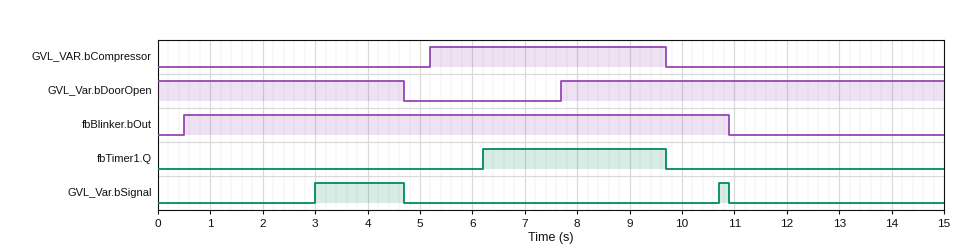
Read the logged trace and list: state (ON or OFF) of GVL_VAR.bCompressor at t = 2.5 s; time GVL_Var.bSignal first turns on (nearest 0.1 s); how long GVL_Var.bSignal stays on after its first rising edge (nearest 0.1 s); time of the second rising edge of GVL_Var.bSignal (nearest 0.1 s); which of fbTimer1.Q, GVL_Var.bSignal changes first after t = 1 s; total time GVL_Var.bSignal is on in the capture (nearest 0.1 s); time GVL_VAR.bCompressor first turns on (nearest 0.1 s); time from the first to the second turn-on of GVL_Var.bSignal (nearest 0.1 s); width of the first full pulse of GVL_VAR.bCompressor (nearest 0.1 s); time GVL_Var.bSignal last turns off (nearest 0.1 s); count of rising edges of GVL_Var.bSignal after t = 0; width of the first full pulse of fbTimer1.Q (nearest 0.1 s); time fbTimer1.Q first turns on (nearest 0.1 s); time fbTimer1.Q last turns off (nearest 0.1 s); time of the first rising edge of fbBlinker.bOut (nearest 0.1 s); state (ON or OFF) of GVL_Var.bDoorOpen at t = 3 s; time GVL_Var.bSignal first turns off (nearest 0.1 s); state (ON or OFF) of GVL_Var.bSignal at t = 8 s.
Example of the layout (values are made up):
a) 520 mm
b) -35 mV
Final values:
a) OFF
b) 3.0 s
c) 1.7 s
d) 10.7 s
e) GVL_Var.bSignal
f) 1.9 s
g) 5.2 s
h) 7.7 s
i) 4.5 s
j) 10.9 s
k) 2
l) 3.5 s
m) 6.2 s
n) 9.7 s
o) 0.5 s
p) ON
q) 4.7 s
r) OFF
